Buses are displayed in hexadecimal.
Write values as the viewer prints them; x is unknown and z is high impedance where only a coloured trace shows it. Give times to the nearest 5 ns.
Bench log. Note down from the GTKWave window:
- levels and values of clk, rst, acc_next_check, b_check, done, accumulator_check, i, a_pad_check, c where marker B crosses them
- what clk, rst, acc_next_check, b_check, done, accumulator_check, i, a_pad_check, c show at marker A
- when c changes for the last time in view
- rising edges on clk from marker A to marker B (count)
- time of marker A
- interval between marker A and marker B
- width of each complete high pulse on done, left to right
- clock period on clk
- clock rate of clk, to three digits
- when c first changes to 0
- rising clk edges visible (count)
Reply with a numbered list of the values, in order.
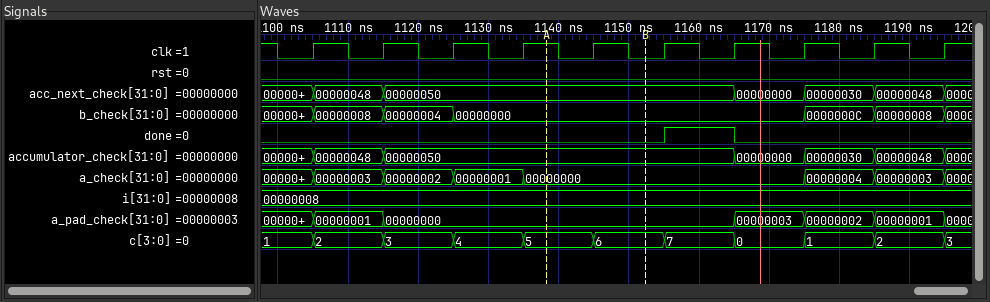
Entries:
1. clk=0, rst=0, acc_next_check=00000050, b_check=00000000, done=0, accumulator_check=00000050, i=00000008, a_pad_check=00000000, c=6
2. clk=1, rst=0, acc_next_check=00000050, b_check=00000000, done=0, accumulator_check=00000050, i=00000008, a_pad_check=00000000, c=5
3. 1195 ns
4. 1
5. 1140 ns
6. 15 ns
7. 10 ns
8. 10 ns
9. 100 MHz
10. 1165 ns
11. 10
